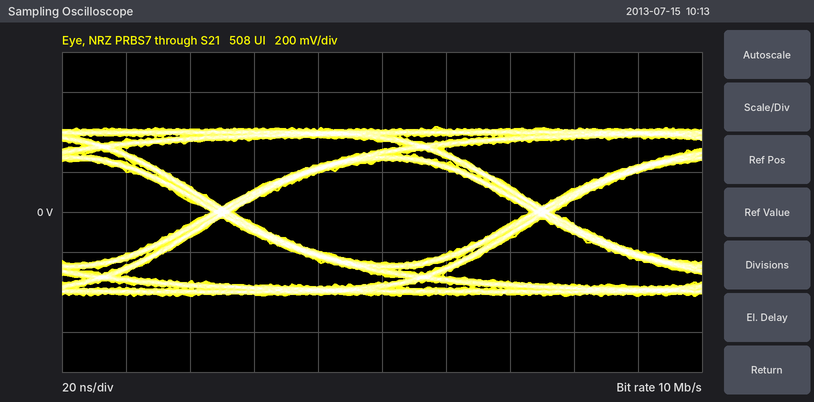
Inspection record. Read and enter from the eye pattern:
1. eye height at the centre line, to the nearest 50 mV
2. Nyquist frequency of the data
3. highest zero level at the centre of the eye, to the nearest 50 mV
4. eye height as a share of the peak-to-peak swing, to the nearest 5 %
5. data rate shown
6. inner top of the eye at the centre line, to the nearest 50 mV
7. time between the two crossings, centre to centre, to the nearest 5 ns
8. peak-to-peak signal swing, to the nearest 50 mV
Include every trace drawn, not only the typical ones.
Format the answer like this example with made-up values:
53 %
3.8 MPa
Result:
500 mV
5 MHz
-250 mV
60 %
10 Mb/s
250 mV
100 ns
850 mV
